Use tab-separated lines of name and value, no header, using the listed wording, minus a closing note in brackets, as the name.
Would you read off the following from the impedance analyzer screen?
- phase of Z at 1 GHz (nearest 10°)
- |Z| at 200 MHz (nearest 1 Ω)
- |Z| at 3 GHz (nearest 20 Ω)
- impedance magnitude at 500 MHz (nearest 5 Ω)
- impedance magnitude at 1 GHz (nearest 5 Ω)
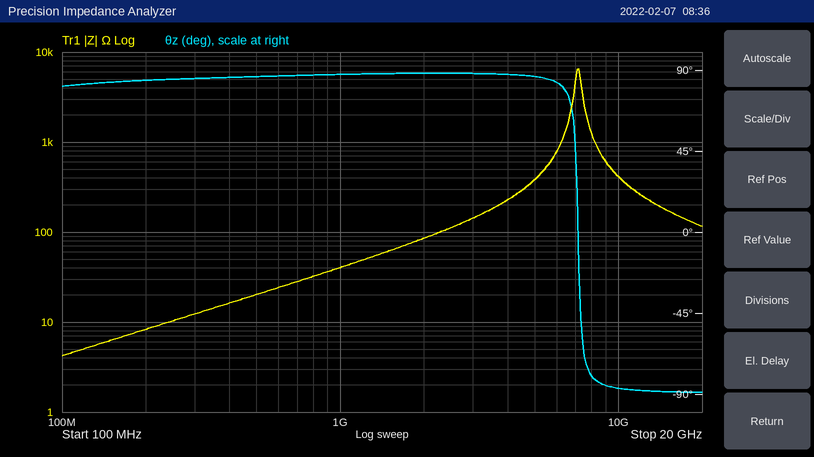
phase of Z at 1 GHz	90°
|Z| at 200 MHz	8 Ω
|Z| at 3 GHz	140 Ω
impedance magnitude at 500 MHz	20 Ω
impedance magnitude at 1 GHz	40 Ω
